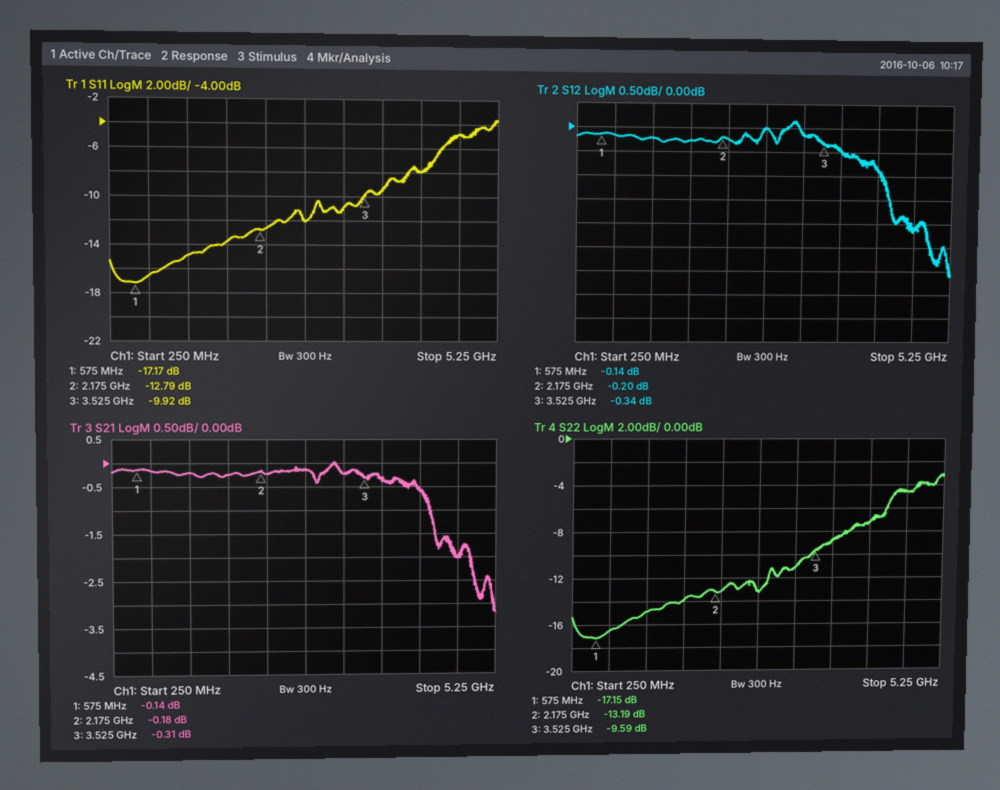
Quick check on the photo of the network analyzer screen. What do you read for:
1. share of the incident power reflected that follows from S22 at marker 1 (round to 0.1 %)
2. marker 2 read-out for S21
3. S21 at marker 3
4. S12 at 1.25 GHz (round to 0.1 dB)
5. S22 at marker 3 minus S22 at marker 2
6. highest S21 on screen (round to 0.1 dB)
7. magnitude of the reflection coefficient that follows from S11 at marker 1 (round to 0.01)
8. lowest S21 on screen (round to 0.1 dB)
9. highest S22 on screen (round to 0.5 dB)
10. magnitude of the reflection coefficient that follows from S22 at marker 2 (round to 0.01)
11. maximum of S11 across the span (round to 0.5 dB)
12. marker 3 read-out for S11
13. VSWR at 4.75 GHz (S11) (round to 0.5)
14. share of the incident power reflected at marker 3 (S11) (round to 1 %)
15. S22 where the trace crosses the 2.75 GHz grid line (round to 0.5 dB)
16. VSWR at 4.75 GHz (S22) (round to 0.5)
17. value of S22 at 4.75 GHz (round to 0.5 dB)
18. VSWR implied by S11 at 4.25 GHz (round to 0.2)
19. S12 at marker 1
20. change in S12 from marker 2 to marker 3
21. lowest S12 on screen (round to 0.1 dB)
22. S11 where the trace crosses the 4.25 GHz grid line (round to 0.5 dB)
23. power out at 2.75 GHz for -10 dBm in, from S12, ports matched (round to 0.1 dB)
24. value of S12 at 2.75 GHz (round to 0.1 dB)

1.9 %
-0.18 dB
-0.31 dB
-0.2 dB
3.60 dB
0.0 dB
0.14
-3.2 dB
-3.0 dB
0.22
-3.5 dB
-9.92 dB
3.5
10 %
-13.0 dB
4.0
-4.5 dB
2.4
-0.14 dB
-0.14 dB
-3.1 dB
-8.0 dB
-10.0 dBm
0.0 dB
